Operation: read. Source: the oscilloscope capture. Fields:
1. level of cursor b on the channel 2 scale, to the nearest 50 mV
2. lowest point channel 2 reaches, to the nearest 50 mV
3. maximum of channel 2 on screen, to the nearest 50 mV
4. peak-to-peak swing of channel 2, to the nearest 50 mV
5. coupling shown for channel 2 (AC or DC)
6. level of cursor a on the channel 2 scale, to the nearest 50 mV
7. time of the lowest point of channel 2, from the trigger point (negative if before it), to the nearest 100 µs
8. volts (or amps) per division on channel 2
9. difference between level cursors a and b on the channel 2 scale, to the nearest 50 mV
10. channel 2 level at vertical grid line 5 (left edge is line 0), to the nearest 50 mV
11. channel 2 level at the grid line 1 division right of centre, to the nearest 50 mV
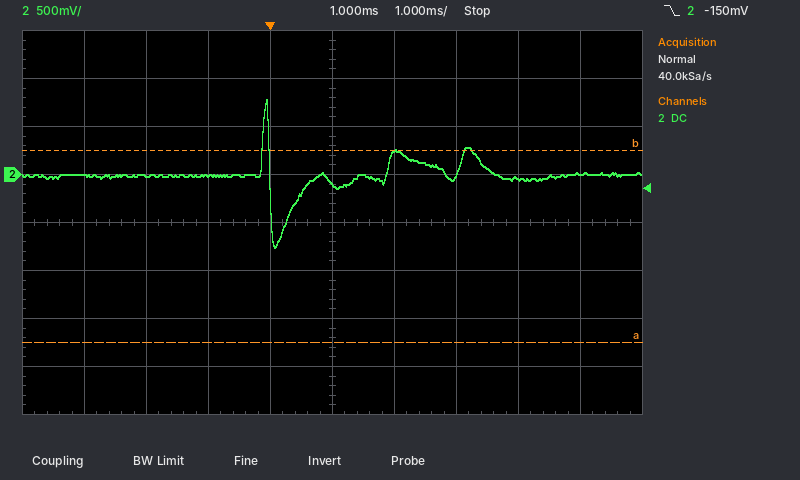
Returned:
250 mV
-750 mV
800 mV
1.55 V
DC
-1.75 V
+100 µs
500 mV
2.00 V
-100 mV
250 mV
